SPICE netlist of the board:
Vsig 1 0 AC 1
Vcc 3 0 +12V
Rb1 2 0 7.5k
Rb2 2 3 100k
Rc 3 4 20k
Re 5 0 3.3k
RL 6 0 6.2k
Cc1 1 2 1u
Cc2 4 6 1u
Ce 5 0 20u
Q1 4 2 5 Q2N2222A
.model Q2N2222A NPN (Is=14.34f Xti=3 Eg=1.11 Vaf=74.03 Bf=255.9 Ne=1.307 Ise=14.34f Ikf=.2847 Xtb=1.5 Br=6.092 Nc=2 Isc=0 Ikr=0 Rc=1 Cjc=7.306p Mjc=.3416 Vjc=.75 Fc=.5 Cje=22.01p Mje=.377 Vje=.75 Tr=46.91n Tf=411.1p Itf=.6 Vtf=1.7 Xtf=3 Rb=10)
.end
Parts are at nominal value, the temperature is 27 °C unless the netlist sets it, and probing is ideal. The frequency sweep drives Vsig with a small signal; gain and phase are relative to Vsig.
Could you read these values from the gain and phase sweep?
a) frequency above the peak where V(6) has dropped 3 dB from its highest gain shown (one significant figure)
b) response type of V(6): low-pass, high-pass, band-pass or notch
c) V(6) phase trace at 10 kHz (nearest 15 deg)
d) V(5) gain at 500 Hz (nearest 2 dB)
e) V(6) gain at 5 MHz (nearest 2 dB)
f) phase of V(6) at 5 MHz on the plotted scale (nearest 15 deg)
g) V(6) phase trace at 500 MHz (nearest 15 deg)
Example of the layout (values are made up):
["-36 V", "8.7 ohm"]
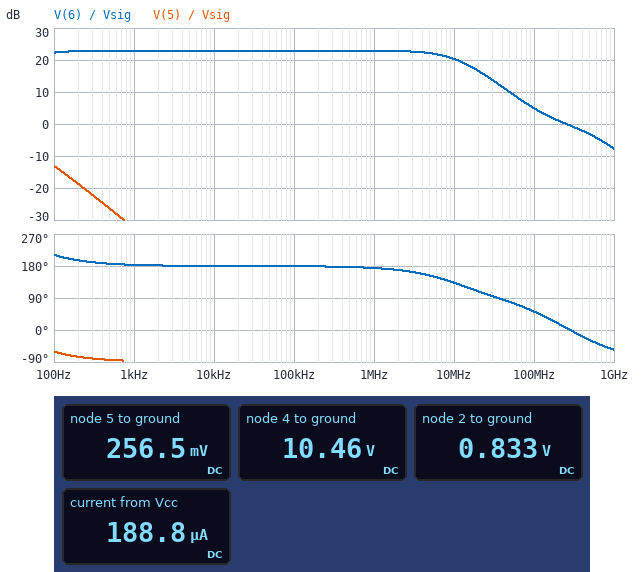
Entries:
["10 MHz", "low-pass", "180 deg", "-26 dB", "22 dB", "150 deg", "-30 deg"]
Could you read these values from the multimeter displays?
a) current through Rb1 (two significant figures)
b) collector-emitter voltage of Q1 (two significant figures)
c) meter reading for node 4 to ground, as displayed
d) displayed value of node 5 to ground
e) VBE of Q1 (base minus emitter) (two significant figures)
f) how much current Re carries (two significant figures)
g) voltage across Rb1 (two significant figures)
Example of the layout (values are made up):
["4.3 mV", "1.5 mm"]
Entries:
["110 µA", "10 V", "10.46 V", "256.5 mV", "580 mV", "78 µA", "830 mV"]
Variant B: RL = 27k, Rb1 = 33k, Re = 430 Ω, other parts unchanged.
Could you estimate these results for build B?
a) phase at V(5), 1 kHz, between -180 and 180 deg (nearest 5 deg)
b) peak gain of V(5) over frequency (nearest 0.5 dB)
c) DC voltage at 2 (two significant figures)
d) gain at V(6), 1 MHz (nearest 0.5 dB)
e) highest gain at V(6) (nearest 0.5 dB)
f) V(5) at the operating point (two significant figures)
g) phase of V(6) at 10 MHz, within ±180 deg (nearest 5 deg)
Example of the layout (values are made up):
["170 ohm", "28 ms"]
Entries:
["-45 deg", "-26.5 dB", "940 mV", "0 dB", "0.5 dB", "290 mV", "40 deg"]
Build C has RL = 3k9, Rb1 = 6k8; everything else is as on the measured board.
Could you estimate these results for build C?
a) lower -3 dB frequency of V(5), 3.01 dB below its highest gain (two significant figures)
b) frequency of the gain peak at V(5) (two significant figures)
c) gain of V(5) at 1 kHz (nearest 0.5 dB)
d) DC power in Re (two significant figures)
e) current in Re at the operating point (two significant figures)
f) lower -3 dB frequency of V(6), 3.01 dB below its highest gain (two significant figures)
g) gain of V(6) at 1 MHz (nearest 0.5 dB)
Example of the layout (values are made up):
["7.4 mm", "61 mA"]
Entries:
["9.0 Hz", "23 Hz", "-35.0 dB", "11 µW", "58 µA", "39 Hz", "17.0 dB"]
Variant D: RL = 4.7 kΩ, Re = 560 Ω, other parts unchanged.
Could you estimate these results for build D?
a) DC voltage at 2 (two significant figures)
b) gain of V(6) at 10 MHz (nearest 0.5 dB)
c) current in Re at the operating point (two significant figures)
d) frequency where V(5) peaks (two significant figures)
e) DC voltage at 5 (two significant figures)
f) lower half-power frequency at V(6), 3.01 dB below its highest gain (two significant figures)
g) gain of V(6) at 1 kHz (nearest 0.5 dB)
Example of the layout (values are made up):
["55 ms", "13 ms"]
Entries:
["820 mV", "31.0 dB", "360 µA", "55 Hz", "200 mV", "140 Hz", "34.0 dB"]
